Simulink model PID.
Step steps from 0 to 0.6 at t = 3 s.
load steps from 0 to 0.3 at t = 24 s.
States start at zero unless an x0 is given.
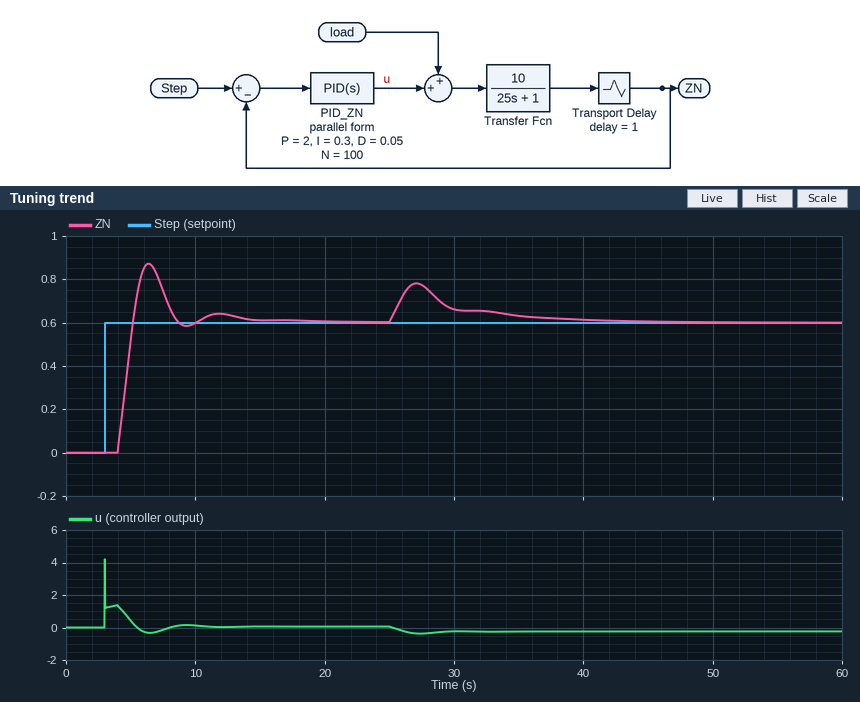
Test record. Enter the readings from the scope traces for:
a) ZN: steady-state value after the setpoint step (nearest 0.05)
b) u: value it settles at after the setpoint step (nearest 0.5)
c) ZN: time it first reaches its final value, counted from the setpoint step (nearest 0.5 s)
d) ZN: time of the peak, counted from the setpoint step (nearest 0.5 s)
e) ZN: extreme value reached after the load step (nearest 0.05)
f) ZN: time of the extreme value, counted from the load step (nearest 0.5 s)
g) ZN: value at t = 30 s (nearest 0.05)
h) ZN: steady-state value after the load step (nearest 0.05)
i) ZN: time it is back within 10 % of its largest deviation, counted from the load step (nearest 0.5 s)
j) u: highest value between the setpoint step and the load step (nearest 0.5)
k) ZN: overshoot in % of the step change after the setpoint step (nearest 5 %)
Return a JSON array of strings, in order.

["0.60", "0.0", "2.0 s", "3.5 s", "0.80", "3.0 s", "0.65", "0.60", "14.5 s", "4.0", "45 %"]
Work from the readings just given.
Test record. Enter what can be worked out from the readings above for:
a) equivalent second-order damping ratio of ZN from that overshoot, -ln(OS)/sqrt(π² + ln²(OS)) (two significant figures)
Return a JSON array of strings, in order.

["0.25"]
